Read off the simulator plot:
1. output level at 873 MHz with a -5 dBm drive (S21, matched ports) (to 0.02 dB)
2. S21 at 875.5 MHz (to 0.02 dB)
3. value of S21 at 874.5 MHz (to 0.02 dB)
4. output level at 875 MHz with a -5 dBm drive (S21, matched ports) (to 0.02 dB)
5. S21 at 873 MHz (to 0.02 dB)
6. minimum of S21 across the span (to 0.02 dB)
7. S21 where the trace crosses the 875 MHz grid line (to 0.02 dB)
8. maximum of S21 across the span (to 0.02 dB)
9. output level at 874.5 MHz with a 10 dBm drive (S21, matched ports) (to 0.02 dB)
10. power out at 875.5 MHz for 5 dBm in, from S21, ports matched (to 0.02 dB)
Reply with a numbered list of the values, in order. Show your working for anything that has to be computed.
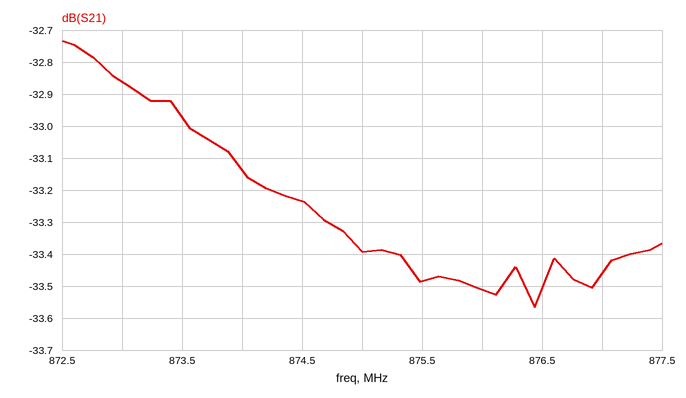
1. -5 dBm + (-32.86 dB) = -37.86 dBm
2. -33.48 dB
3. -33.24 dB
4. -5 dBm + (-33.40 dB) = -38.40 dBm
5. -32.86 dB
6. -33.56 dB
7. -33.40 dB
8. -32.74 dB
9. 10 dBm + (-33.24 dB) = -23.24 dBm
10. 5 dBm + (-33.48 dB) = -28.48 dBm
